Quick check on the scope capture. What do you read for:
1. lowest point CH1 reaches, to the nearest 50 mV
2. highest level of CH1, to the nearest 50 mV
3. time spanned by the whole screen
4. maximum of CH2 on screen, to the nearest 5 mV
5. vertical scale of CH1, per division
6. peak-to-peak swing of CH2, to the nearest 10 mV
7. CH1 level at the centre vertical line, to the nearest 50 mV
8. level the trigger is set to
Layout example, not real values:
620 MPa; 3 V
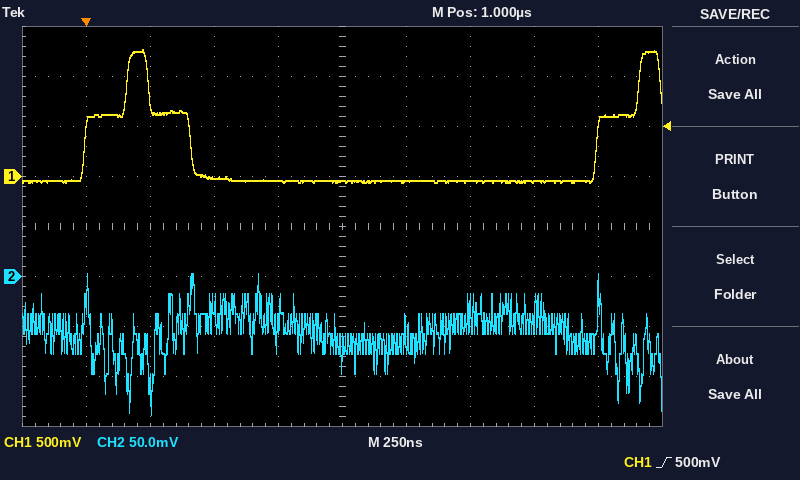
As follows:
-50 mV; 1.25 V; 2.5 µs; 5 mV; 500 mV; 140 mV; -50 mV; 500 mV
